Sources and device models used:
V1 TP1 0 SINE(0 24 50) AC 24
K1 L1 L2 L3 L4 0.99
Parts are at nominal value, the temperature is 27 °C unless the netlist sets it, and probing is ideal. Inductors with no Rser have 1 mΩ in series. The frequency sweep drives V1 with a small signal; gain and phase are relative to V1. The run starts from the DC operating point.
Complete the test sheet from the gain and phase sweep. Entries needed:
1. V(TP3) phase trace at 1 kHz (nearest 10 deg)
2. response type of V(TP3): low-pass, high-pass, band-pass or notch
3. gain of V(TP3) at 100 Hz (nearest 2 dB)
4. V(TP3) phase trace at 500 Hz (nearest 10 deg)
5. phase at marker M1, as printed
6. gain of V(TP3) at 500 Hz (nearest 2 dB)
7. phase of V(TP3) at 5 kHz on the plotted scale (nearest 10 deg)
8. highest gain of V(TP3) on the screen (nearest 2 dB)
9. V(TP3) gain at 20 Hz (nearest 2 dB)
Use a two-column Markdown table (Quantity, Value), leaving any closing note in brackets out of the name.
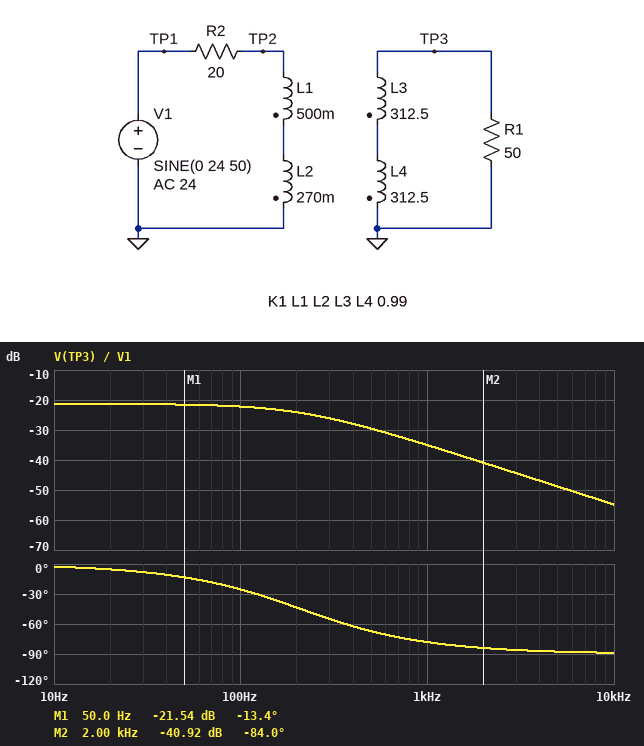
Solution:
| Quantity | Value |
|---|---|
| V(TP3) phase trace at 1 kHz | -80 deg |
| response type of V(TP3): low-pass, high-pass, band-pass or notch | low-pass |
| gain of V(TP3) at 100 Hz | -22 dB |
| V(TP3) phase trace at 500 Hz | -70 deg |
| phase at marker M1, as printed | -13.4 deg |
| gain of V(TP3) at 500 Hz | -30 dB |
| phase of V(TP3) at 5 kHz on the plotted scale | -90 deg |
| highest gain of V(TP3) on the screen | -22 dB |
| V(TP3) gain at 20 Hz | -22 dB |
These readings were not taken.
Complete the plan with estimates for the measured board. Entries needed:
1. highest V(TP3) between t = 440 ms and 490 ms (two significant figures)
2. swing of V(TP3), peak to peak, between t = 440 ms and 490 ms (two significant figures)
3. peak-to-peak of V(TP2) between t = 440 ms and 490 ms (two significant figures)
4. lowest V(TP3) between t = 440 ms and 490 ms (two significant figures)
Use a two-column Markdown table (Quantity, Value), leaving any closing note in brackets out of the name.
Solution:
| Quantity | Value |
|---|---|
| highest V(TP3) between t = 440 ms and 490 ms | 2.0 V |
| swing of V(TP3), peak to peak, between t = 440 ms and 490 ms | 4.0 V |
| peak-to-peak of V(TP2) between t = 440 ms and 490 ms | 11 V |
| lowest V(TP3) between t = 440 ms and 490 ms | -2.0 V |
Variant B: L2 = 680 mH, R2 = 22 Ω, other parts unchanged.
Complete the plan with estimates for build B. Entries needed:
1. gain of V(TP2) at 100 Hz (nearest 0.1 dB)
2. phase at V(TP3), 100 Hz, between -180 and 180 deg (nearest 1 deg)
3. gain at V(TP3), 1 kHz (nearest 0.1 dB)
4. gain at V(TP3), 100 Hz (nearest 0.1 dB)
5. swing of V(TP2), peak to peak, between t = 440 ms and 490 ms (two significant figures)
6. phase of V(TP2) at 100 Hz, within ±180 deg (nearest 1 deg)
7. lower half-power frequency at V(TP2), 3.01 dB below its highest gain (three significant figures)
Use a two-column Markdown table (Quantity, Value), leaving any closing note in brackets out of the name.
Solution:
| Quantity | Value |
|---|---|
| gain of V(TP2) at 100 Hz | -5.1 dB |
| phase at V(TP3), 100 Hz, between -180 and 180 deg | -34 deg |
| gain at V(TP3), 1 kHz | -36.8 dB |
| gain at V(TP3), 100 Hz | -21.8 dB |
| swing of V(TP2), peak to peak, between t = 440 ms and 490 ms | 15 V |
| phase of V(TP2) at 100 Hz, within ±180 deg | 56 deg |
| lower half-power frequency at V(TP2), 3.01 dB below its highest gain | 150 Hz |
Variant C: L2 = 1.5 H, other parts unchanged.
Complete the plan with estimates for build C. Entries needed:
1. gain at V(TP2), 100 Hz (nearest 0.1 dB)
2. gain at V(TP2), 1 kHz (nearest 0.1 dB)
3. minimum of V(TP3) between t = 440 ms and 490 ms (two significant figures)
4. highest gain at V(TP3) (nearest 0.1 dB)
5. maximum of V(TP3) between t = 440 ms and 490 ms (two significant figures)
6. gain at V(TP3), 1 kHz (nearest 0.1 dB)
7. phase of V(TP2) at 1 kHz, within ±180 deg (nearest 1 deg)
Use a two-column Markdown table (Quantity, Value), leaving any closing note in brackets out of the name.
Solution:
| Quantity | Value |
|---|---|
| gain at V(TP2), 100 Hz | -2.3 dB |
| gain at V(TP2), 1 kHz | 0 dB |
| minimum of V(TP3) between t = 440 ms and 490 ms | -2.8 V |
| highest gain at V(TP3) | -17.4 dB |
| maximum of V(TP3) between t = 440 ms and 490 ms | 2.8 V |
| gain at V(TP3), 1 kHz | -39.0 dB |
| phase of V(TP2) at 1 kHz, within ±180 deg | 5 deg |
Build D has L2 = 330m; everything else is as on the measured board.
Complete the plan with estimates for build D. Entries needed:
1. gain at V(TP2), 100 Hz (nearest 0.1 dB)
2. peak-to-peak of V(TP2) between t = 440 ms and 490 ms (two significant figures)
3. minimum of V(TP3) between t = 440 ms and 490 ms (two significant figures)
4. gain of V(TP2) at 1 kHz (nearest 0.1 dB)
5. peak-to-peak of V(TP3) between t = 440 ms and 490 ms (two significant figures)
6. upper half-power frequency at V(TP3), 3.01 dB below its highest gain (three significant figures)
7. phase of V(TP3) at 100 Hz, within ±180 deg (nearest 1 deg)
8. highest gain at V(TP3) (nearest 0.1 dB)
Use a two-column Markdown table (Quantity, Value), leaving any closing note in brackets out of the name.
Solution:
| Quantity | Value |
|---|---|
| gain at V(TP2), 100 Hz | -6.8 dB |
| peak-to-peak of V(TP2) between t = 440 ms and 490 ms | 12 V |
| minimum of V(TP3) between t = 440 ms and 490 ms | -2.1 V |
| gain of V(TP2) at 1 kHz | -0.2 dB |
| peak-to-peak of V(TP3) between t = 440 ms and 490 ms | 4.2 V |
| upper half-power frequency at V(TP3), 3.01 dB below its highest gain | 194 Hz |
| phase of V(TP3) at 100 Hz, within ±180 deg | -27 deg |
| highest gain at V(TP3) | -20.9 dB |
